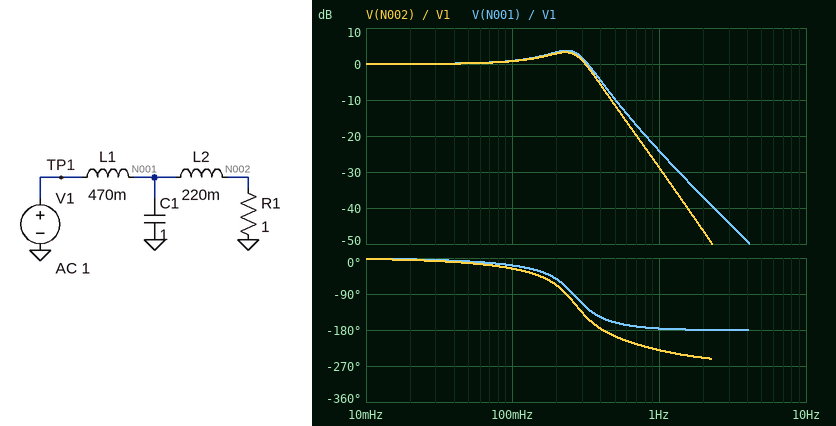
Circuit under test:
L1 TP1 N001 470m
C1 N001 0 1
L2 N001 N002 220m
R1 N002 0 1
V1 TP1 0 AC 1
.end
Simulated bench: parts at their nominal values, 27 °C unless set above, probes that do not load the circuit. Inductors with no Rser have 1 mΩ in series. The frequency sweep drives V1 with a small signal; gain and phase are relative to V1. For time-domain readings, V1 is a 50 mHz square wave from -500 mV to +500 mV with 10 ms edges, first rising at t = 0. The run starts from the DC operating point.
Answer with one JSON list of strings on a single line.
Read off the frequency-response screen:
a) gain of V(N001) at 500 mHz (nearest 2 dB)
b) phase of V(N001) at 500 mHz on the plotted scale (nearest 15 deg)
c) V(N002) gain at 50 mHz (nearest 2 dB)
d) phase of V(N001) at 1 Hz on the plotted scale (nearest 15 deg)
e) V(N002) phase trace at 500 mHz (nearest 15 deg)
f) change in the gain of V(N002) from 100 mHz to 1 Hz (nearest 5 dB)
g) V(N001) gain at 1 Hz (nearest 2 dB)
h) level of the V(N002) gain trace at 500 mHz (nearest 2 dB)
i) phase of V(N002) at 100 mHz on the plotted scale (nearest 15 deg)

["-10 dB", "-165 deg", "0 dB", "-180 deg", "-195 deg", "-30 dB", "-24 dB", "-12 dB", "-30 deg"]
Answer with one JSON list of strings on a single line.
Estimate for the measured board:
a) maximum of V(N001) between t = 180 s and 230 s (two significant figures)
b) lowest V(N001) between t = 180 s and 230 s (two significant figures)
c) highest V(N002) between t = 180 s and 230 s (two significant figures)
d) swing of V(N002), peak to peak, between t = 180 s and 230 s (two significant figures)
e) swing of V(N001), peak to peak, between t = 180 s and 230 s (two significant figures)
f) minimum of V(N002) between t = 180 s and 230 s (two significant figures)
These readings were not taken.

["810 mV", "-810 mV", "790 mV", "1.6 V", "1.6 V", "-790 mV"]
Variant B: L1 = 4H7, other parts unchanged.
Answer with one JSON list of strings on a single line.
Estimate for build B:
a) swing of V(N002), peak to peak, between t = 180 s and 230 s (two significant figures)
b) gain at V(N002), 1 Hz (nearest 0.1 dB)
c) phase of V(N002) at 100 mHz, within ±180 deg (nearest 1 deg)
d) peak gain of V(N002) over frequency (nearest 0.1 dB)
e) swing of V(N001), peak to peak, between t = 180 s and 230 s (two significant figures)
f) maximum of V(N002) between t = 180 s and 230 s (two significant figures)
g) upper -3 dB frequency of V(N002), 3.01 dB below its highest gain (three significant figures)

["820 mV", "-49.3 dB", "-107 deg", "0 dB", "830 mV", "410 mV", "40.4 mHz"]
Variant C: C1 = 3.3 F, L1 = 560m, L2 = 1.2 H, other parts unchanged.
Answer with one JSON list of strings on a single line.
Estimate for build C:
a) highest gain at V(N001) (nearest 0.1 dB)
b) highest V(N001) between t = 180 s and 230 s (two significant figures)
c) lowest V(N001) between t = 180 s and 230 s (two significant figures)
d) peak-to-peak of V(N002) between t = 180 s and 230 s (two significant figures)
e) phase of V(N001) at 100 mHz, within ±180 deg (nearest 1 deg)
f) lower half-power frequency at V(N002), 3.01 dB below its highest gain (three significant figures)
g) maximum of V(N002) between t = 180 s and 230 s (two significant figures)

["12.6 dB", "1.1 V", "-1.1 V", "1.8 V", "-27 deg", "113 mHz", "920 mV"]
